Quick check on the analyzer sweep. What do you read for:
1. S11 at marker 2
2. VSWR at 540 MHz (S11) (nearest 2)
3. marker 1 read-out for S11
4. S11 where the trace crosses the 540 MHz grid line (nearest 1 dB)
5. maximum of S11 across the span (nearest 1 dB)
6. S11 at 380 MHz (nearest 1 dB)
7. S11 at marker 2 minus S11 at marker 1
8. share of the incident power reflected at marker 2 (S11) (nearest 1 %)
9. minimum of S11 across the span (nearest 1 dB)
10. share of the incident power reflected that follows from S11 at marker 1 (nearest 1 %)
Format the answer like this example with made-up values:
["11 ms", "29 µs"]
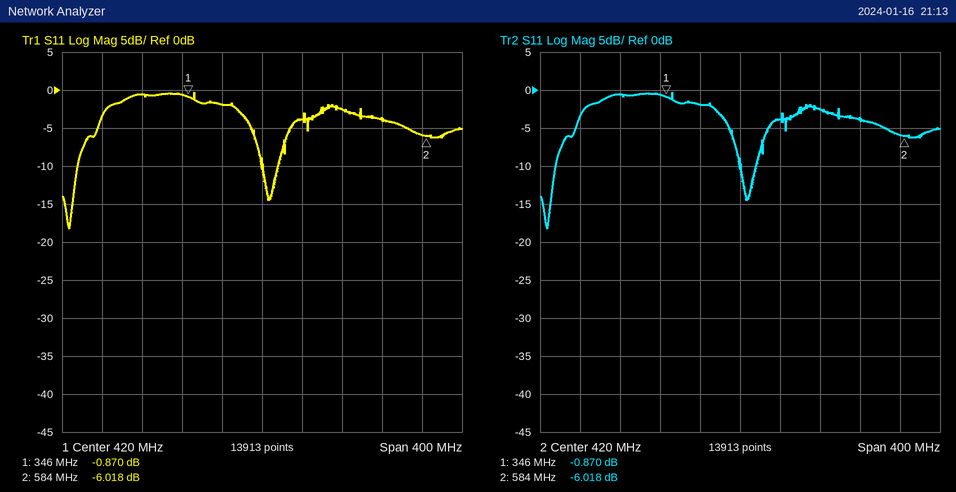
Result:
["-6.018 dB", "4", "-0.870 dB", "-4 dB", "0 dB", "-2 dB", "-5.148 dB", "25 %", "-18 dB", "82 %"]
